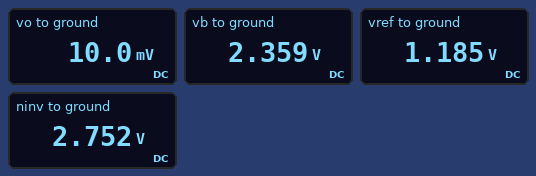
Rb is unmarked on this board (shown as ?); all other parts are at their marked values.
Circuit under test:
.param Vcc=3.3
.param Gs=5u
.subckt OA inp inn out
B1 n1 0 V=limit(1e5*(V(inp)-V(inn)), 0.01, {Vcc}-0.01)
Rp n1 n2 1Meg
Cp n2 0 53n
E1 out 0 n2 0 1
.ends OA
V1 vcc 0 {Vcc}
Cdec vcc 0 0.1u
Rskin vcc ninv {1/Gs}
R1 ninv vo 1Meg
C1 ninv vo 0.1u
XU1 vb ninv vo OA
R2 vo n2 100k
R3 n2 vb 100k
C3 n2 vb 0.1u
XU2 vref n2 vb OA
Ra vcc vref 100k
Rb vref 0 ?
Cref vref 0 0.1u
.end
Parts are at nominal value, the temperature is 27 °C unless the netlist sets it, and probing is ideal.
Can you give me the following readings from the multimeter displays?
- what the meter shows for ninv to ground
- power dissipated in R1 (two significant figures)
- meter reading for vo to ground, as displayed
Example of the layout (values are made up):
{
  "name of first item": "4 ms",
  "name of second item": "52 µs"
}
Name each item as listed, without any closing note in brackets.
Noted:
{
  "what the meter shows for ninv to ground": "2.752 V",
  "power dissipated in R1": "7.5 µW",
  "meter reading for vo to ground, as displayed": "10.0 mV"
}
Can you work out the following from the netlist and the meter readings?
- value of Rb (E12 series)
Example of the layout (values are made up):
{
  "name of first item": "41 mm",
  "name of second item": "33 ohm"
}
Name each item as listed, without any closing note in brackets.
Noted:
{
  "value of Rb": "56 kΩ"
}
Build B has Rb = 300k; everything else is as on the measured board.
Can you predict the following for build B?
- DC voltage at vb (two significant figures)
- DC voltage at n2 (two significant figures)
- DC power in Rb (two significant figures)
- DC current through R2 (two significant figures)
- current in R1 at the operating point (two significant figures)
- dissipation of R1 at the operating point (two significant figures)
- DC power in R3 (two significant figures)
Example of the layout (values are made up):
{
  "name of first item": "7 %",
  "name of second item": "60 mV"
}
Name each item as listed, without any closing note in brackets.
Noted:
{
  "DC voltage at vb": "3.1 V",
  "DC voltage at n2": "2.5 V",
  "DC power in Rb": "20 µW",
  "DC current through R2": "5.9 µA",
  "current in R1 at the operating point": "1.2 µA",
  "dissipation of R1 at the operating point": "1.4 µW",
  "DC power in R3": "3.5 µW"
}
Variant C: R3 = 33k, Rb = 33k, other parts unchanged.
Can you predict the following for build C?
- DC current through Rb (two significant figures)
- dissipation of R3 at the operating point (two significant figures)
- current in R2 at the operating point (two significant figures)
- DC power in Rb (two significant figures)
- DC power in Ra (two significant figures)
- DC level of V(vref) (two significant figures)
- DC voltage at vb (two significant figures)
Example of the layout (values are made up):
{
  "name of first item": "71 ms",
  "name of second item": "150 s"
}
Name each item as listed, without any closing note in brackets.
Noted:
{
  "DC current through Rb": "25 µA",
  "dissipation of R3 at the operating point": "2.2 µW",
  "current in R2 at the operating point": "8.1 µA",
  "DC power in Rb": "20 µW",
  "DC power in Ra": "62 µW",
  "DC level of V(vref)": "820 mV",
  "DC voltage at vb": "1.1 V"
}
